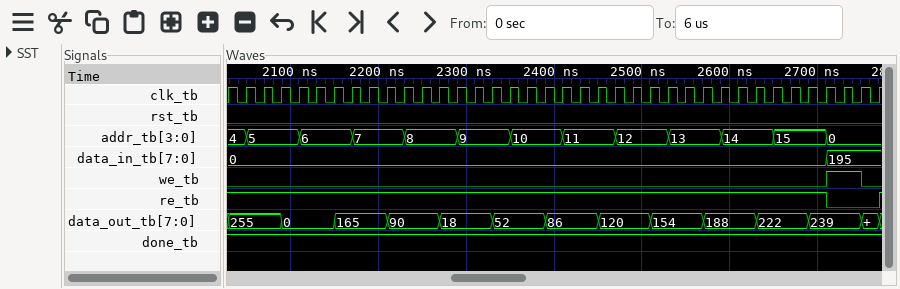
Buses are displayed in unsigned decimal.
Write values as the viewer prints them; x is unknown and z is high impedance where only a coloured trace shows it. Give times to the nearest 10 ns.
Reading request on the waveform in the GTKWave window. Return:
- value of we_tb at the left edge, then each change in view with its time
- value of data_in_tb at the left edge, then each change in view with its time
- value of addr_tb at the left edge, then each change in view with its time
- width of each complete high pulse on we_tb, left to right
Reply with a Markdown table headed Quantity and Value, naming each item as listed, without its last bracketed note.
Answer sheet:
| Quantity | Value |
|---|---|
| value of we_tb at the left edge, then each change in view with its time | 0, 1 at 2710 ns, 0 at 2750 ns |
| value of data_in_tb at the left edge, then each change in view with its time | 0, 195 at 2710 ns |
| value of addr_tb at the left edge, then each change in view with its time | 4, 5 at 2050 ns, 6 at 2110 ns, 7 at 2170 ns, 8 at 2230 ns, 9 at 2290 ns, 10 at 2350 ns, 11 at 2410 ns, 12 at 2470 ns, 13 at 2530 ns, 14 at 2590 ns, 15 at 2650 ns, 0 at 2710 ns |
| width of each complete high pulse on we_tb, left to right | 40 ns |
